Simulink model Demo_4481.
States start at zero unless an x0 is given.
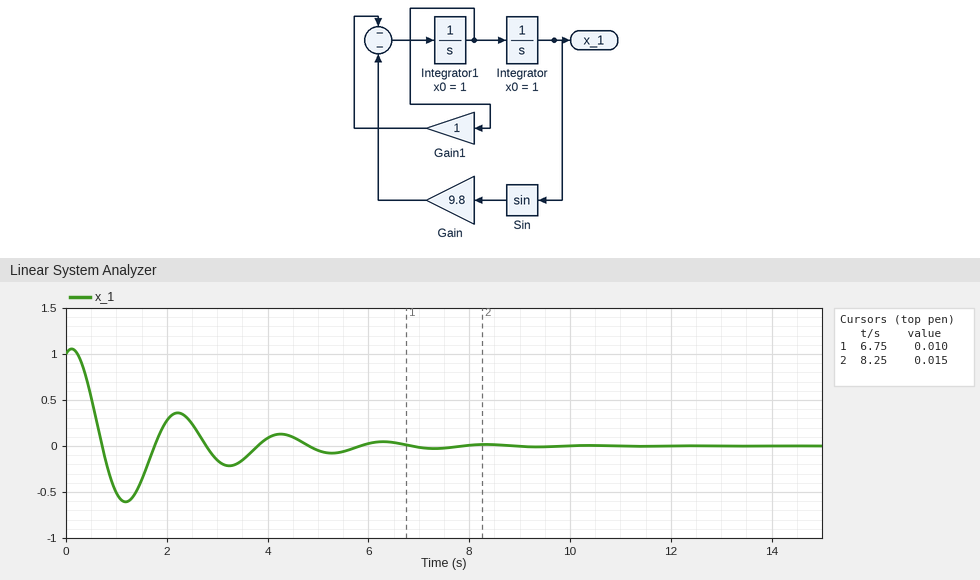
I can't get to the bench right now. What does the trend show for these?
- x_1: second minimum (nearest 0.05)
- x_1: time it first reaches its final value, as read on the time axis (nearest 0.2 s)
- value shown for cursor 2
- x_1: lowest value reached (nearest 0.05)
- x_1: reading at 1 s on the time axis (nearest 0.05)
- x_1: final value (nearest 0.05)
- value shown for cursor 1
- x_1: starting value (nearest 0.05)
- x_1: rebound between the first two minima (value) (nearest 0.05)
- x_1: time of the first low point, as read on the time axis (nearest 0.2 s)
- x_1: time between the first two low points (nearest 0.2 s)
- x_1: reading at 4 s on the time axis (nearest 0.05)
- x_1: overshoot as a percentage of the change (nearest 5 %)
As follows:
-0.20
0.8 s
0.015
-0.60
-0.50
0.00
0.010
1.00
0.35
1.2 s
2.0 s
0.10
60 %
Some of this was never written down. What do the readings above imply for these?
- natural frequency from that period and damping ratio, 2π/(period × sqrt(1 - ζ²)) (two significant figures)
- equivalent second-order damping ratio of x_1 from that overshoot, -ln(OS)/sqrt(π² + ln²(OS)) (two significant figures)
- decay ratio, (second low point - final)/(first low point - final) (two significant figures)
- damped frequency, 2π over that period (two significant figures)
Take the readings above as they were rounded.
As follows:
3.2 rad/s
0.16
0.33
3.1 rad/s
